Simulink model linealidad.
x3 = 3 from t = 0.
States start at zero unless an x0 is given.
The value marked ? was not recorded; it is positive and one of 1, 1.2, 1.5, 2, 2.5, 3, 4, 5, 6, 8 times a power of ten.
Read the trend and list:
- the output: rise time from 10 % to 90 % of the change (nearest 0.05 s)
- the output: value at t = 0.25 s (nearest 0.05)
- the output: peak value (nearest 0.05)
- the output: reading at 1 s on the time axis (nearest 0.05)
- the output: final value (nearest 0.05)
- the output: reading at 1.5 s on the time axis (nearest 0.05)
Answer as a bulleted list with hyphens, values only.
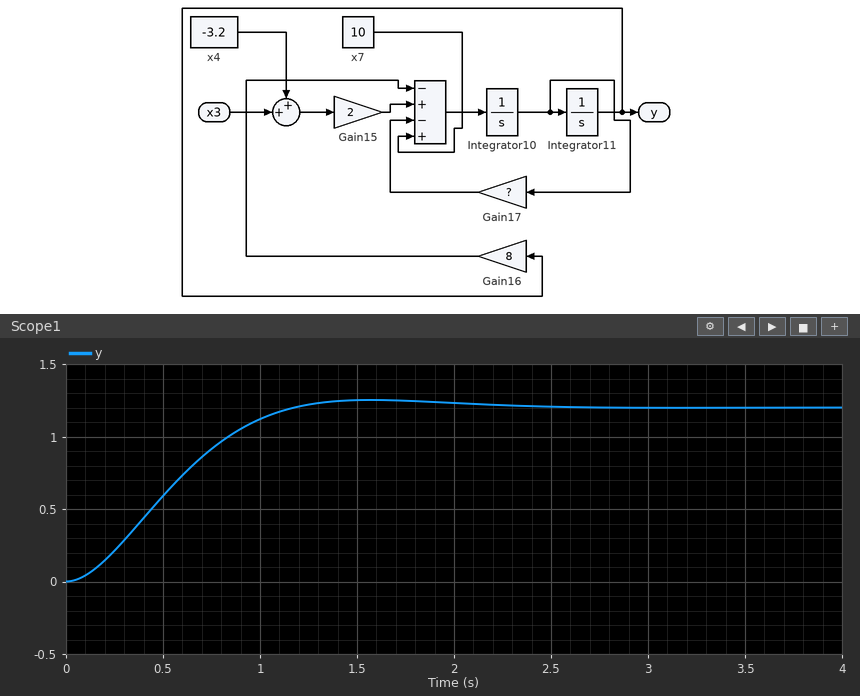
- 0.75 s
- 0.20
- 1.25
- 1.10
- 1.20
- 1.25
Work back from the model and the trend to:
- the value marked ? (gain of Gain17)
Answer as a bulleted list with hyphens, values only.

- 4
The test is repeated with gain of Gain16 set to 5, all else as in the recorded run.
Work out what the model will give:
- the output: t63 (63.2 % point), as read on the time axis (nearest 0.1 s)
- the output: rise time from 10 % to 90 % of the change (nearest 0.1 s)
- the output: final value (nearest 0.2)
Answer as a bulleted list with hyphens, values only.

- 0.9 s
- 1.3 s
- 2.0
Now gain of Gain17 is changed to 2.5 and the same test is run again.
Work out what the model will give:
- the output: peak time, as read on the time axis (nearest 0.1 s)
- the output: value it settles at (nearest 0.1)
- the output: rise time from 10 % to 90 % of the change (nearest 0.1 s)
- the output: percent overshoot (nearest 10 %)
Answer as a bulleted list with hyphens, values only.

- 1.2 s
- 1.2
- 0.5 s
- 20 %
